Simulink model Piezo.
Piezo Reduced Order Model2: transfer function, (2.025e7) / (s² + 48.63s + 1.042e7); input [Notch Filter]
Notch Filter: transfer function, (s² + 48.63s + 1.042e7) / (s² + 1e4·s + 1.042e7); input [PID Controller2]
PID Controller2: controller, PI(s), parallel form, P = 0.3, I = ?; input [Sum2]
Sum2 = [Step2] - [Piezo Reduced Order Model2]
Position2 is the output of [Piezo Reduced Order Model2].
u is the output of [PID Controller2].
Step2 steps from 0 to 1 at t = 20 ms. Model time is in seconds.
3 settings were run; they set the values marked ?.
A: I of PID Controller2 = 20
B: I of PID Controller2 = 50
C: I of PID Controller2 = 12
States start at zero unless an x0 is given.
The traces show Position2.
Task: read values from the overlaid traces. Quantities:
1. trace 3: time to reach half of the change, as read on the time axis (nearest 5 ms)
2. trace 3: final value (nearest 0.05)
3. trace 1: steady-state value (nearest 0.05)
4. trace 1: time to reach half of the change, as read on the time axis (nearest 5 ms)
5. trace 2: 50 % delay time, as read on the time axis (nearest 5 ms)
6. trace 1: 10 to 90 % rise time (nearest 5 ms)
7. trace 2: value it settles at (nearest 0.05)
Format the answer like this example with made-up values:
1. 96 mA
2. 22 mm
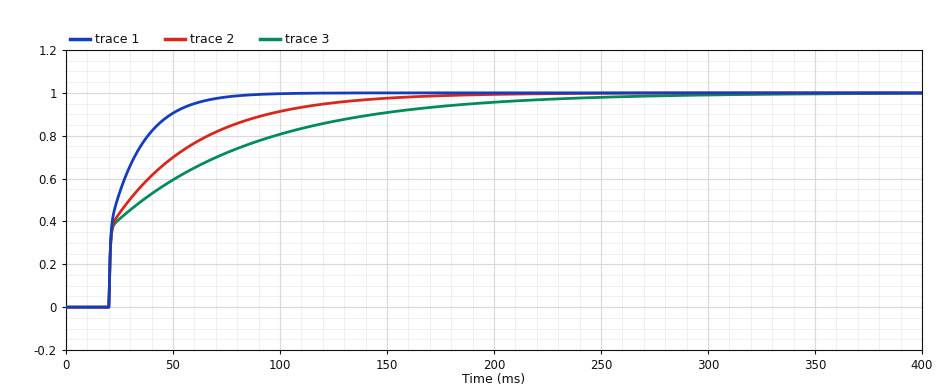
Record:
1. 35 ms
2. 1.00
3. 1.00
4. 25 ms
5. 30 ms
6. 30 ms
7. 1.00
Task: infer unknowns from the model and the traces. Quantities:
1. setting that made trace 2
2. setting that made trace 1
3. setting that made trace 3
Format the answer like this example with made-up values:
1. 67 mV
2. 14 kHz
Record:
1. A
2. B
3. C
